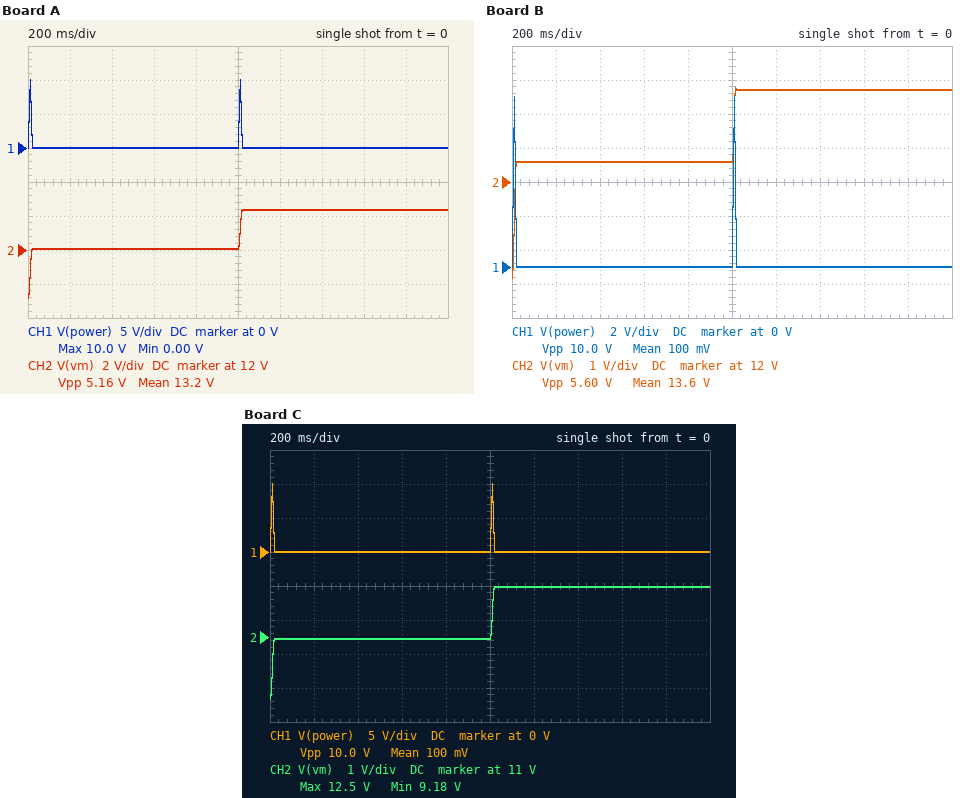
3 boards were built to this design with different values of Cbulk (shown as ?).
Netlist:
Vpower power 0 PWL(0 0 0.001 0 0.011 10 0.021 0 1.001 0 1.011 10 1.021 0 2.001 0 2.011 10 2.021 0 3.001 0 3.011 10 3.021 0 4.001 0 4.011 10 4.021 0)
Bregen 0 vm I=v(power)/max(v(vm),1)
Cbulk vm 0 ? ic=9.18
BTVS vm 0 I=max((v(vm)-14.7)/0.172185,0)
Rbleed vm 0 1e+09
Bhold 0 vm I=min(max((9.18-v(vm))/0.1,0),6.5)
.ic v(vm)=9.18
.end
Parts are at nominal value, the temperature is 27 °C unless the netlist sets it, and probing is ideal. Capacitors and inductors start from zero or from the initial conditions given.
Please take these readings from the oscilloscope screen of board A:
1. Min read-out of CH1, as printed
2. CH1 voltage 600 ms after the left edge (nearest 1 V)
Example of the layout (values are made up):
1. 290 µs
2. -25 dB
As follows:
1. 0.00 V
2. 0 V
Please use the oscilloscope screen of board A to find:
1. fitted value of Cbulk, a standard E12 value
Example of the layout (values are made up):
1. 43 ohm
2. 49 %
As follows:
1. 3.3 mF
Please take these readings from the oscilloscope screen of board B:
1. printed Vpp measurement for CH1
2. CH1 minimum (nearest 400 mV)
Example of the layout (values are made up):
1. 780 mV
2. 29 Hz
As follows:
1. 10.0 V
2. 0 V
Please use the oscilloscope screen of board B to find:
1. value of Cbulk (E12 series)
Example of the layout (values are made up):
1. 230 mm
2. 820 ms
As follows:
1. 2.7 mF
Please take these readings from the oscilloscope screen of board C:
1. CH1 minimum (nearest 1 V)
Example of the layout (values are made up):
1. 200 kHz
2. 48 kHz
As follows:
1. 0 V
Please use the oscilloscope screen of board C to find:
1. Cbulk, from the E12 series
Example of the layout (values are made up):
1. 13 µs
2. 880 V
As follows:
1. 5.6 mF
